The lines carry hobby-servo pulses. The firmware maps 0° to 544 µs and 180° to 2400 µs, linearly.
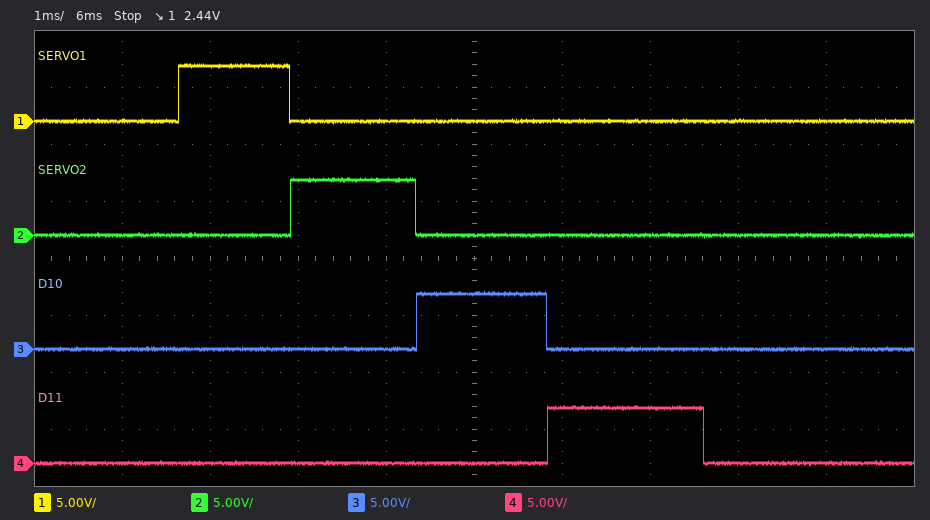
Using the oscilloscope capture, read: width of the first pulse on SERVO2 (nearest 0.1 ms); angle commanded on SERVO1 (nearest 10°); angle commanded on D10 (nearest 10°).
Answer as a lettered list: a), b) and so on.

a) 1.4 ms
b) 70°
c) 90°
